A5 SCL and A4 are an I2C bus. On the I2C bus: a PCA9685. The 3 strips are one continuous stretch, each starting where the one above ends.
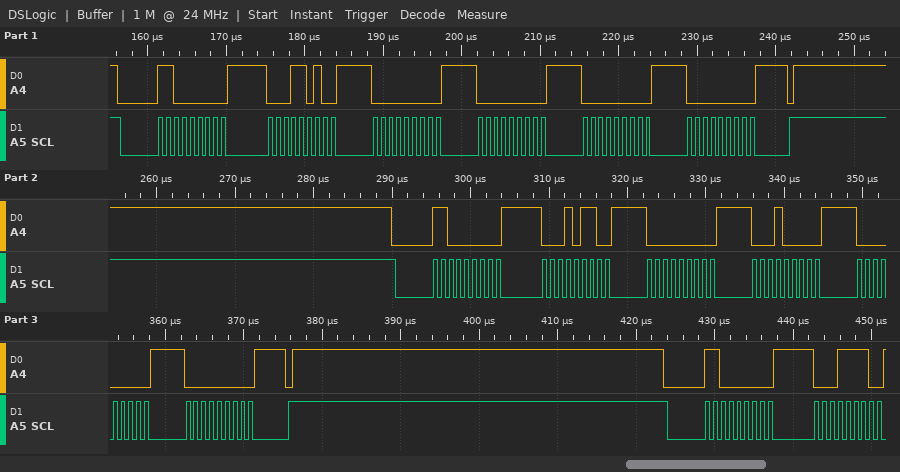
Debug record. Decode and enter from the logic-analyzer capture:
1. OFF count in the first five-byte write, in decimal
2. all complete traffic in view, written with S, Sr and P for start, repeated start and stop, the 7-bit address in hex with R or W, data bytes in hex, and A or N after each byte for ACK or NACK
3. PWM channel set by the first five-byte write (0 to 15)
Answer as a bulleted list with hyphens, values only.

- 0
- S 60W A 1A A 00 A 00 A 00 A 00 A P S 60W A 16 A 00 A 10 A 00 A 00 A P S 60W A 1E A
- 5
